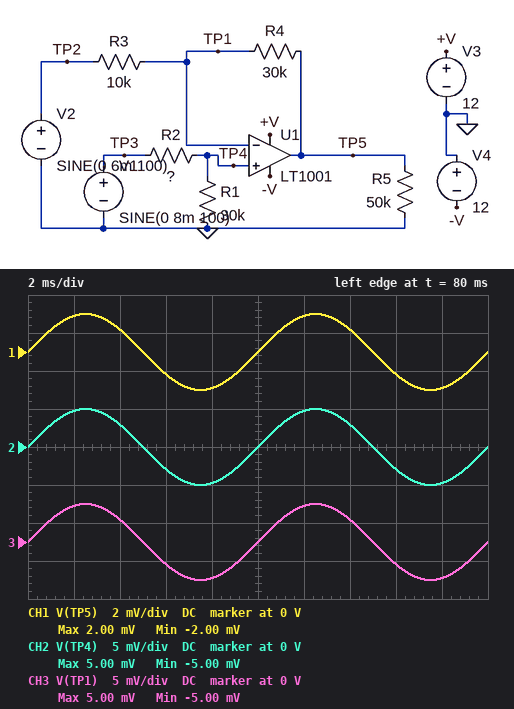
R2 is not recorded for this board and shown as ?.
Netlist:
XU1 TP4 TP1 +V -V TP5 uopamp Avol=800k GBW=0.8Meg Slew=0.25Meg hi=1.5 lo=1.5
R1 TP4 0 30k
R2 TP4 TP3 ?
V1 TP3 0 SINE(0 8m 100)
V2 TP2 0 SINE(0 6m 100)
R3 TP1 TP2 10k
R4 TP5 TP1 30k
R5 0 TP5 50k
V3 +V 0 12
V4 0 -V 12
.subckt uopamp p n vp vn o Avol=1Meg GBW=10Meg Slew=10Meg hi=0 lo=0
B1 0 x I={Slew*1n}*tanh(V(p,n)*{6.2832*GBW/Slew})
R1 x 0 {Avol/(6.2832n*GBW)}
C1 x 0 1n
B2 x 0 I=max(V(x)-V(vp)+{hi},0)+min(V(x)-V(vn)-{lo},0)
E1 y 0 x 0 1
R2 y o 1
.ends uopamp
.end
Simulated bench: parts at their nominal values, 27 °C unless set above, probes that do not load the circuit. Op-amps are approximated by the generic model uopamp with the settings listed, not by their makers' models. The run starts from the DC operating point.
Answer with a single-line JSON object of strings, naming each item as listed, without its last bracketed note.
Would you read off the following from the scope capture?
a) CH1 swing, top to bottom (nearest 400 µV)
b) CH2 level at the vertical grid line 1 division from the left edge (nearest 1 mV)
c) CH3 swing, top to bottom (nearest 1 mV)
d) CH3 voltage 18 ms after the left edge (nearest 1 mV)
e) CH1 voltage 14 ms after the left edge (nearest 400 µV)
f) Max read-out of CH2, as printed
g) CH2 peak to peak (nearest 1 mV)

{"CH1 swing, top to bottom": "4.0 mV", "CH2 level at the vertical grid line 1 division from the left edge": "5 mV", "CH3 swing, top to bottom": "10 mV", "CH3 voltage 18 ms after the left edge": "-5 mV", "CH1 voltage 14 ms after the left edge": "1.2 mV", "Max read-out of CH2, as printed": "5.00 mV", "CH2 peak to peak": "10 mV"}
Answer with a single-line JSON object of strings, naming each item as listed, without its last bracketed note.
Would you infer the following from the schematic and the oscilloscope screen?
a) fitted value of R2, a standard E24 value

{"fitted value of R2, a standard E24 value": "18 kΩ"}
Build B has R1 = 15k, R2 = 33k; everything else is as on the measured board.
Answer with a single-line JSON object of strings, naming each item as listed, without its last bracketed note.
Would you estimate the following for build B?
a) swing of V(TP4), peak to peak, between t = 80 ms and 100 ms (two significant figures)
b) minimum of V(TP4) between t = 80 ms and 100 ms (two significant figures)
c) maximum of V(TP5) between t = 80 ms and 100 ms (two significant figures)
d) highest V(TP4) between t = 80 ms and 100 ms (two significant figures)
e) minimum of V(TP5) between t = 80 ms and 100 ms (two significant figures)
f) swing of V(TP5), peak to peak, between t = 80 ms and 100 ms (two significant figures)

{"swing of V(TP4), peak to peak, between t = 80 ms and 100 ms": "5.0 mV", "minimum of V(TP4) between t = 80 ms and 100 ms": "-2.5 mV", "maximum of V(TP5) between t = 80 ms and 100 ms": "8.0 mV", "highest V(TP4) between t = 80 ms and 100 ms": "2.5 mV", "minimum of V(TP5) between t = 80 ms and 100 ms": "-8.0 mV", "swing of V(TP5), peak to peak, between t = 80 ms and 100 ms": "16 mV"}
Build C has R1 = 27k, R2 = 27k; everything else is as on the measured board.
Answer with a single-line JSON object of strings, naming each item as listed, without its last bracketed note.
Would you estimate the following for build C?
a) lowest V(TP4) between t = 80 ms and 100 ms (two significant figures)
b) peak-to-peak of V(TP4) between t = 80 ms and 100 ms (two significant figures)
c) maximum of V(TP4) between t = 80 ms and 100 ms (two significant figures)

{"lowest V(TP4) between t = 80 ms and 100 ms": "-4.0 mV", "peak-to-peak of V(TP4) between t = 80 ms and 100 ms": "8.0 mV", "maximum of V(TP4) between t = 80 ms and 100 ms": "4.0 mV"}
